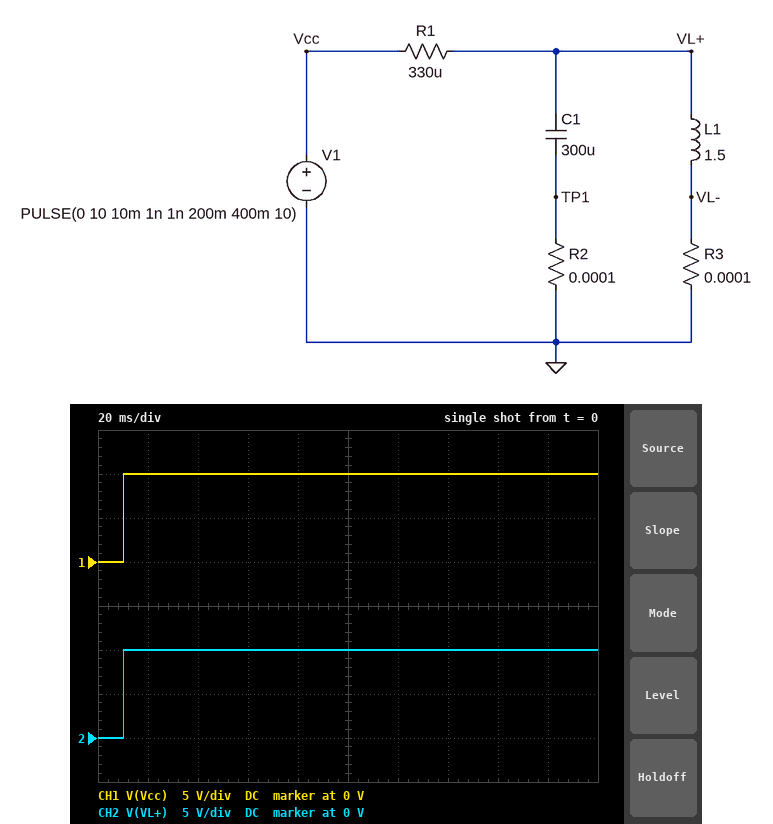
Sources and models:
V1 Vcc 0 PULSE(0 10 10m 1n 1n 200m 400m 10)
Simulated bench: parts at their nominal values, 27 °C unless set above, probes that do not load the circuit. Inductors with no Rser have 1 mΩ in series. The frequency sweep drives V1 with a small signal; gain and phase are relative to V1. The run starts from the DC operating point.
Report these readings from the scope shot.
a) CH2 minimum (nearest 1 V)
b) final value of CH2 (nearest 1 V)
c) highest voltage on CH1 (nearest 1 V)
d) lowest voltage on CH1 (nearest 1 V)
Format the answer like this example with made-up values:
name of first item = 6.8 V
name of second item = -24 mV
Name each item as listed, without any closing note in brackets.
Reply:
CH2 minimum = 0 V
final value of CH2 = 10 V
highest voltage on CH1 = 10 V
lowest voltage on CH1 = 0 V
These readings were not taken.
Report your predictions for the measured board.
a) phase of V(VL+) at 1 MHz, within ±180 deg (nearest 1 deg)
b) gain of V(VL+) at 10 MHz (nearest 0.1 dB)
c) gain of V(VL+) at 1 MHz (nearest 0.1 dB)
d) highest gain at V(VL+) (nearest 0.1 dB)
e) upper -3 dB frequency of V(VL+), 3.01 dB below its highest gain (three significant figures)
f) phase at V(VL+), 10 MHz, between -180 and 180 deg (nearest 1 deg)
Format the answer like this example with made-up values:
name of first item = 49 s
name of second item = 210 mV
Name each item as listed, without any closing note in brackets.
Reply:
phase of V(VL+) at 1 MHz, within ±180 deg = -28 deg
gain of V(VL+) at 10 MHz = -11.7 dB
gain of V(VL+) at 1 MHz = -2.0 dB
highest gain at V(VL+) = 0 dB
upper -3 dB frequency of V(VL+), 3.01 dB below its highest gain = 1.31 MHz
phase at V(VL+), 10 MHz, between -180 and 180 deg = -21 deg
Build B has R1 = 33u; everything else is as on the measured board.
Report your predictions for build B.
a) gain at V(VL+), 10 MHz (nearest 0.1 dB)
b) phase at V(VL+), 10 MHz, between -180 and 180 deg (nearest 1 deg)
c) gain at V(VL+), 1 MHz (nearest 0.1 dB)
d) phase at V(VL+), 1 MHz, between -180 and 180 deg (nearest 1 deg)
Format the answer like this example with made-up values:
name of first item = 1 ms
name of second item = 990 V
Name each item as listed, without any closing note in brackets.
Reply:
gain at V(VL+), 10 MHz = -2.0 dB
phase at V(VL+), 10 MHz, between -180 and 180 deg = -6 deg
gain at V(VL+), 1 MHz = -0.1 dB
phase at V(VL+), 1 MHz, between -180 and 180 deg = -3 deg
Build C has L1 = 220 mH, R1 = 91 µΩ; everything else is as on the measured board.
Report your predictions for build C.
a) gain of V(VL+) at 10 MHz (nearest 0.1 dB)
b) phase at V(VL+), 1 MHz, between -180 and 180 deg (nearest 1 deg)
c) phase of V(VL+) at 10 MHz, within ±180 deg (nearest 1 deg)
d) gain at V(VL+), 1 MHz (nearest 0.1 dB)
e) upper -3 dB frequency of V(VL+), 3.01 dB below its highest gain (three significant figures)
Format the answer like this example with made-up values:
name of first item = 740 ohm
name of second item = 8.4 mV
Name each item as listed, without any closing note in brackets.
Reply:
gain of V(VL+) at 10 MHz = -4.9 dB
phase at V(VL+), 1 MHz, between -180 and 180 deg = -9 deg
phase of V(VL+) at 10 MHz, within ±180 deg = -12 deg
gain at V(VL+), 1 MHz = -0.4 dB
upper -3 dB frequency of V(VL+), 3.01 dB below its highest gain = 4.13 MHz
